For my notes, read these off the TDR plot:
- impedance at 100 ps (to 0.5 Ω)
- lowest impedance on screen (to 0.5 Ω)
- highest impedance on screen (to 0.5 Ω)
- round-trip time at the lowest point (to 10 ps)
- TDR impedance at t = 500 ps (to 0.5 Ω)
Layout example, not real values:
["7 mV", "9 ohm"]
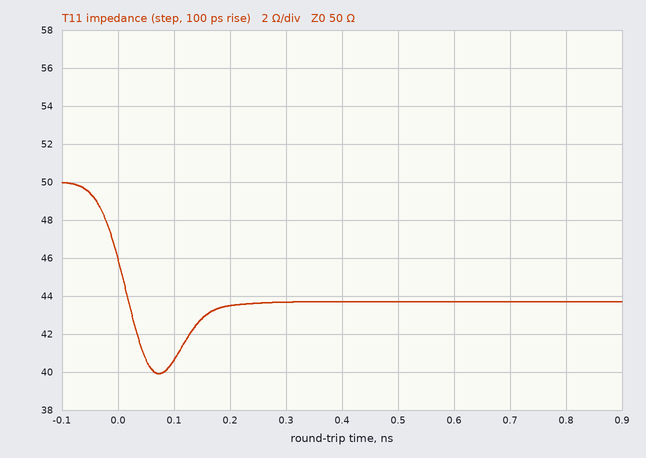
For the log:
["40.5 Ω", "40.0 Ω", "50.0 Ω", "70 ps", "43.5 Ω"]
